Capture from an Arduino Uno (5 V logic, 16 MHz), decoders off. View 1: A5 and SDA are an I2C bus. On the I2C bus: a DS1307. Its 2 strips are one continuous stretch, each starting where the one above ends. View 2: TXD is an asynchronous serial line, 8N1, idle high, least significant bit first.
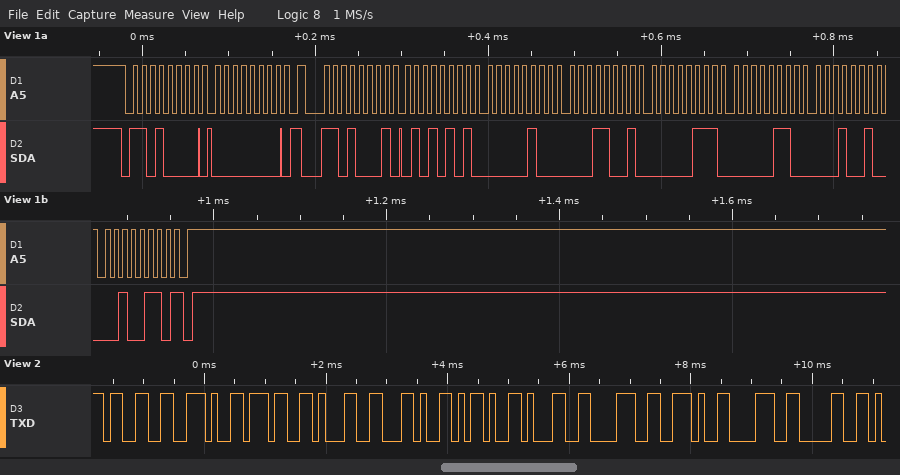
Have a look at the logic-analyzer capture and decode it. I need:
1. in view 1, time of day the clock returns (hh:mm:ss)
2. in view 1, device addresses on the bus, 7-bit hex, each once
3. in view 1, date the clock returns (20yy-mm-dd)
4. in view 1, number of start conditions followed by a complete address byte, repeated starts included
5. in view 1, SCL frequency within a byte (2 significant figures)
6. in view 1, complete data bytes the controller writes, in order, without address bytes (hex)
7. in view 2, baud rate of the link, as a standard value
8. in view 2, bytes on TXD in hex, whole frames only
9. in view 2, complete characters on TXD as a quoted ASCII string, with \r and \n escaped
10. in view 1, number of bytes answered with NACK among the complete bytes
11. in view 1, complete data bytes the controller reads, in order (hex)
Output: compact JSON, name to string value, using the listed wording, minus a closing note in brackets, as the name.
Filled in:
{"in view 1, time of day the clock returns": "19:04:55", "in view 1, device addresses on the bus, 7-bit hex, each once": "0x68", "in view 1, date the clock returns": "2026-12-06", "in view 1, number of start conditions followed by a complete address byte, repeated starts included": "2", "in view 1, SCL frequency within a byte": "100 kHz", "in view 1, complete data bytes the controller writes, in order, without address bytes": "00", "in view 2, baud rate of the link, as a standard value": "9600 baud", "in view 2, bytes on TXD in hex, whole frames only": "33 2E 37 31 2C 2D 31 38 2E 38 30", "in view 2, complete characters on TXD as a quoted ASCII string, with \\r and \\n escaped": "\"3.71,-18.80\"", "in view 1, number of bytes answered with NACK among the complete bytes": "1", "in view 1, complete data bytes the controller reads, in order": "55 04 19 07 06 12 26"}
